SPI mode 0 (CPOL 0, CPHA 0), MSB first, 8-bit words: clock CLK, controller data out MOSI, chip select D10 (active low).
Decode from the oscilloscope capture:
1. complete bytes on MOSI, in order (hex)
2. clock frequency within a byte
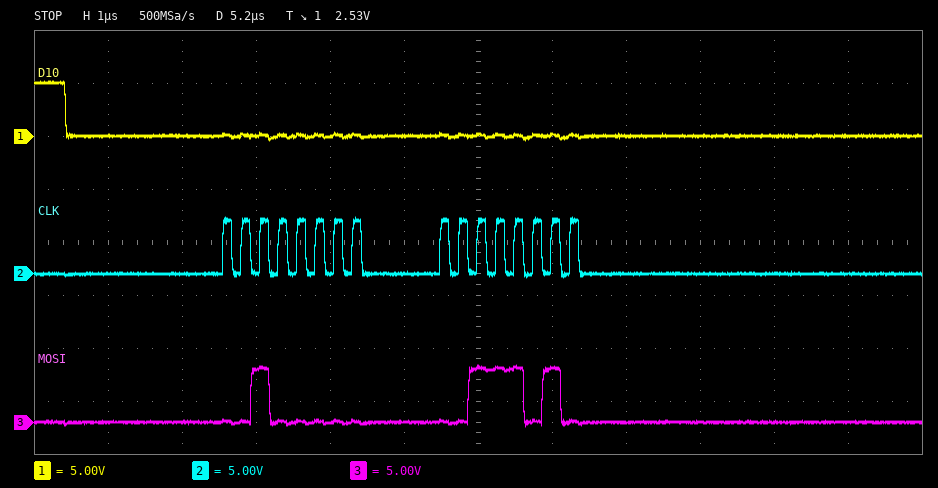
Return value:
20 3A
4 MHz
